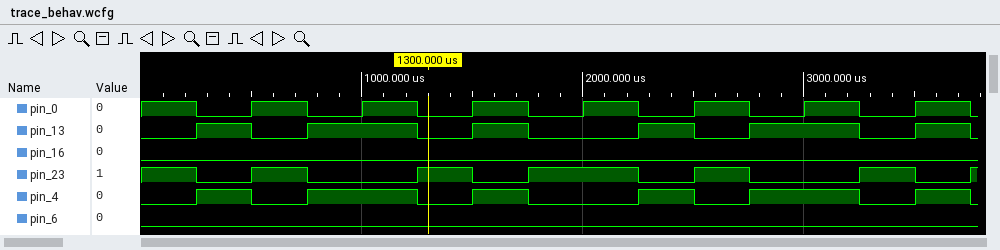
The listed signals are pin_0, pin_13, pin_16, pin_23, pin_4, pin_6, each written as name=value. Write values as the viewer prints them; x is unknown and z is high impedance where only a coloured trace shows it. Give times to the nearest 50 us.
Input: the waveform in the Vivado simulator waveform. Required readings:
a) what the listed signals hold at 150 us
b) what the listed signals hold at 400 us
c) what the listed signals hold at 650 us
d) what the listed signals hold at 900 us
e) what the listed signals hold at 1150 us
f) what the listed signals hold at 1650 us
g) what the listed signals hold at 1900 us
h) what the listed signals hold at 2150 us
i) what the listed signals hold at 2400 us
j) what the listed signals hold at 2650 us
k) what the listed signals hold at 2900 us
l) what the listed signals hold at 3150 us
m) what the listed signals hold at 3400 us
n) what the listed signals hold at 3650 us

pin_0=1, pin_13=0, pin_16=0, pin_23=1, pin_4=0, pin_6=0
pin_0=0, pin_13=1, pin_16=0, pin_23=0, pin_4=1, pin_6=0
pin_0=1, pin_13=0, pin_16=0, pin_23=1, pin_4=0, pin_6=0
pin_0=0, pin_13=1, pin_16=0, pin_23=0, pin_4=1, pin_6=0
pin_0=1, pin_13=1, pin_16=0, pin_23=0, pin_4=1, pin_6=0
pin_0=1, pin_13=1, pin_16=0, pin_23=0, pin_4=1, pin_6=0
pin_0=0, pin_13=0, pin_16=0, pin_23=1, pin_4=0, pin_6=0
pin_0=1, pin_13=0, pin_16=0, pin_23=1, pin_4=0, pin_6=0
pin_0=0, pin_13=1, pin_16=0, pin_23=0, pin_4=1, pin_6=0
pin_0=1, pin_13=0, pin_16=0, pin_23=1, pin_4=0, pin_6=0
pin_0=0, pin_13=1, pin_16=0, pin_23=0, pin_4=1, pin_6=0
pin_0=1, pin_13=1, pin_16=0, pin_23=0, pin_4=1, pin_6=0
pin_0=0, pin_13=0, pin_16=0, pin_23=1, pin_4=0, pin_6=0
pin_0=1, pin_13=1, pin_16=0, pin_23=0, pin_4=1, pin_6=0
